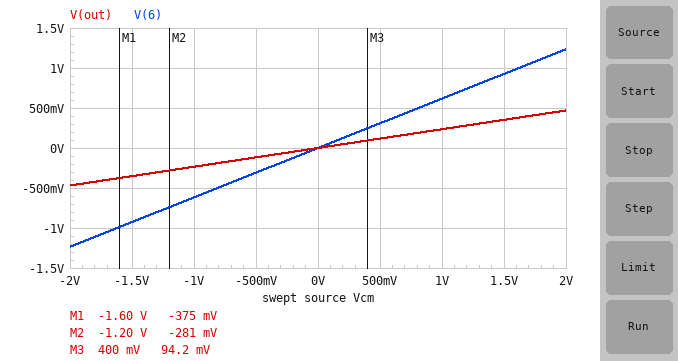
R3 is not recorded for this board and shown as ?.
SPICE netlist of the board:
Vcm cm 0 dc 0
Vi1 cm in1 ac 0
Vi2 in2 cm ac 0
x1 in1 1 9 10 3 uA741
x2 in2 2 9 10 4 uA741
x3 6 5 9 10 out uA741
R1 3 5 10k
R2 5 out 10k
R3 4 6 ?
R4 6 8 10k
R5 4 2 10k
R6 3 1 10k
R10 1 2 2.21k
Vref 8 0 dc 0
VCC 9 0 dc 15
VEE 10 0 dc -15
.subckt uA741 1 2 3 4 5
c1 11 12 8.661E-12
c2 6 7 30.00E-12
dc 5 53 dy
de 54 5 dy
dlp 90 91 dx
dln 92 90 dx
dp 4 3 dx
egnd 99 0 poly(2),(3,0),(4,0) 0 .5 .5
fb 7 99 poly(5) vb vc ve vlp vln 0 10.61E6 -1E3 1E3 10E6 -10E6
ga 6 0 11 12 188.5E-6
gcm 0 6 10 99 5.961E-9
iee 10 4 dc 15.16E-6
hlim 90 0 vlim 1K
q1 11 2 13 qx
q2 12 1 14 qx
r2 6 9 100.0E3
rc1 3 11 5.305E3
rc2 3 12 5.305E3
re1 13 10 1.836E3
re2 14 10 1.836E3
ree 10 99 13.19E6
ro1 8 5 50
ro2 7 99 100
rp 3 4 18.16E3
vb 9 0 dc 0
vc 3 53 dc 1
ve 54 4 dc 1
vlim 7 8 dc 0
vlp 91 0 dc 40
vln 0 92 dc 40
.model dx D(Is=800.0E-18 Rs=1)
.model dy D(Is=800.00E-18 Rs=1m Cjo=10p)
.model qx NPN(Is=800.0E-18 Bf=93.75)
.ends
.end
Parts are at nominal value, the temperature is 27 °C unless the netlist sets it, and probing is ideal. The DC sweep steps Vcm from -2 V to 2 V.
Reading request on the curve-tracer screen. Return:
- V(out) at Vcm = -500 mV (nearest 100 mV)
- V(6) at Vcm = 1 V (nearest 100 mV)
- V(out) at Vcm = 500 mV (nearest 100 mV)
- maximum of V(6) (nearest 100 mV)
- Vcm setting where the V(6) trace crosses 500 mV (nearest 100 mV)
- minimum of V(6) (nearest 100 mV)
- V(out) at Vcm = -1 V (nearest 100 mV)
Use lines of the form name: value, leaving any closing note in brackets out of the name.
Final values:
V(out) at Vcm = -500 mV: -100 mV
V(6) at Vcm = 1 V: 600 mV
V(out) at Vcm = 500 mV: 100 mV
maximum of V(6): 1.2 V
Vcm setting where the V(6) trace crosses 500 mV: 800 mV
minimum of V(6): -1.2 V
V(out) at Vcm = -1 V: -200 mV
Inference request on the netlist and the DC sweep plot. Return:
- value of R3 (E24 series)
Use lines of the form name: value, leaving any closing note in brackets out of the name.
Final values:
value of R3: 6.2 kΩ
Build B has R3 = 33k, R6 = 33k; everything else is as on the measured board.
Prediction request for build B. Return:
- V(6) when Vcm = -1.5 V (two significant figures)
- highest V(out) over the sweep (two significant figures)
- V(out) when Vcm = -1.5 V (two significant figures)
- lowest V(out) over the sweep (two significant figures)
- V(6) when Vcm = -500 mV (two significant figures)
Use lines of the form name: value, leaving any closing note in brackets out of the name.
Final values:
V(6) when Vcm = -1.5 V: -350 mV
highest V(out) over the sweep: 1.1 V
V(out) when Vcm = -1.5 V: 800 mV
lowest V(out) over the sweep: -1.1 V
V(6) when Vcm = -500 mV: -120 mV
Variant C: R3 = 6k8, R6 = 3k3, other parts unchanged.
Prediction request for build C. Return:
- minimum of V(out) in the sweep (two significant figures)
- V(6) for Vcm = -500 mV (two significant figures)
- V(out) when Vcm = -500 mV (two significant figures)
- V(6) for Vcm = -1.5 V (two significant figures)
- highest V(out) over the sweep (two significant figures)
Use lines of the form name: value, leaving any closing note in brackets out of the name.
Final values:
minimum of V(out) in the sweep: -380 mV
V(6) for Vcm = -500 mV: -300 mV
V(out) when Vcm = -500 mV: -94 mV
V(6) for Vcm = -1.5 V: -890 mV
highest V(out) over the sweep: 380 mV
